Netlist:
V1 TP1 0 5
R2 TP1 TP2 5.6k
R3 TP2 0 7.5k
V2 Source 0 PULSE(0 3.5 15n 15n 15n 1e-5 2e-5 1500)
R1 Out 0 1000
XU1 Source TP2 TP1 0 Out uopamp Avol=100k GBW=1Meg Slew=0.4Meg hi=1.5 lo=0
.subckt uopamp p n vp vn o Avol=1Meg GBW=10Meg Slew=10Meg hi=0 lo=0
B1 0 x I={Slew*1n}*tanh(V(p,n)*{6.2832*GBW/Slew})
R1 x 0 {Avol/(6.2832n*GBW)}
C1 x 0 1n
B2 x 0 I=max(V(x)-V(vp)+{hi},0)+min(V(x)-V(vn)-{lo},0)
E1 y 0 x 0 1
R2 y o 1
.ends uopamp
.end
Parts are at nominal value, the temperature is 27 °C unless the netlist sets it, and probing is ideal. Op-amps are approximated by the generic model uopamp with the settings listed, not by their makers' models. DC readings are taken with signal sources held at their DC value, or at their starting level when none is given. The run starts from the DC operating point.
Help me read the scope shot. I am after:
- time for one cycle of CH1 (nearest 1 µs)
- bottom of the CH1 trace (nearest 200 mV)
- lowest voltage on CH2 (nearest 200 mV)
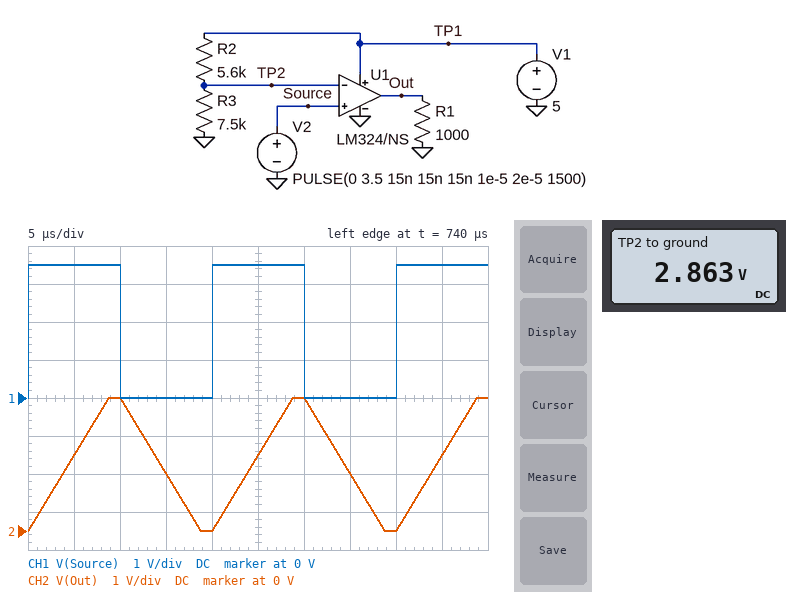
20 µs
0 V
0 V
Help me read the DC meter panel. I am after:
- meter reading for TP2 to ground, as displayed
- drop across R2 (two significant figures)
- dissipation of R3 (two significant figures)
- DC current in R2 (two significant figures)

2.863 V
2.1 V
1.1 mW
380 µA
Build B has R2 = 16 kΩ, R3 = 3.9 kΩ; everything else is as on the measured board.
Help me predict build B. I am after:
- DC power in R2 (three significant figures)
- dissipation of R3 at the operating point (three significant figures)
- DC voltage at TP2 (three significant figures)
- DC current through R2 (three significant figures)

1.01 mW
246 µW
980 mV
251 µA
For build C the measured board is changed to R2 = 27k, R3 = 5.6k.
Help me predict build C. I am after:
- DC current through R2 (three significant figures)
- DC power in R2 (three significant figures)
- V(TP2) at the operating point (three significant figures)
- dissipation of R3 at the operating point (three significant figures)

153 µA
635 µW
859 mV
132 µW
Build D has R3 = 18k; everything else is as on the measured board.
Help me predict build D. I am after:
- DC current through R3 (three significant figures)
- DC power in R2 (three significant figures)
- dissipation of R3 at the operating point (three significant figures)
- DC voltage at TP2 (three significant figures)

212 µA
251 µW
808 µW
3.81 V
